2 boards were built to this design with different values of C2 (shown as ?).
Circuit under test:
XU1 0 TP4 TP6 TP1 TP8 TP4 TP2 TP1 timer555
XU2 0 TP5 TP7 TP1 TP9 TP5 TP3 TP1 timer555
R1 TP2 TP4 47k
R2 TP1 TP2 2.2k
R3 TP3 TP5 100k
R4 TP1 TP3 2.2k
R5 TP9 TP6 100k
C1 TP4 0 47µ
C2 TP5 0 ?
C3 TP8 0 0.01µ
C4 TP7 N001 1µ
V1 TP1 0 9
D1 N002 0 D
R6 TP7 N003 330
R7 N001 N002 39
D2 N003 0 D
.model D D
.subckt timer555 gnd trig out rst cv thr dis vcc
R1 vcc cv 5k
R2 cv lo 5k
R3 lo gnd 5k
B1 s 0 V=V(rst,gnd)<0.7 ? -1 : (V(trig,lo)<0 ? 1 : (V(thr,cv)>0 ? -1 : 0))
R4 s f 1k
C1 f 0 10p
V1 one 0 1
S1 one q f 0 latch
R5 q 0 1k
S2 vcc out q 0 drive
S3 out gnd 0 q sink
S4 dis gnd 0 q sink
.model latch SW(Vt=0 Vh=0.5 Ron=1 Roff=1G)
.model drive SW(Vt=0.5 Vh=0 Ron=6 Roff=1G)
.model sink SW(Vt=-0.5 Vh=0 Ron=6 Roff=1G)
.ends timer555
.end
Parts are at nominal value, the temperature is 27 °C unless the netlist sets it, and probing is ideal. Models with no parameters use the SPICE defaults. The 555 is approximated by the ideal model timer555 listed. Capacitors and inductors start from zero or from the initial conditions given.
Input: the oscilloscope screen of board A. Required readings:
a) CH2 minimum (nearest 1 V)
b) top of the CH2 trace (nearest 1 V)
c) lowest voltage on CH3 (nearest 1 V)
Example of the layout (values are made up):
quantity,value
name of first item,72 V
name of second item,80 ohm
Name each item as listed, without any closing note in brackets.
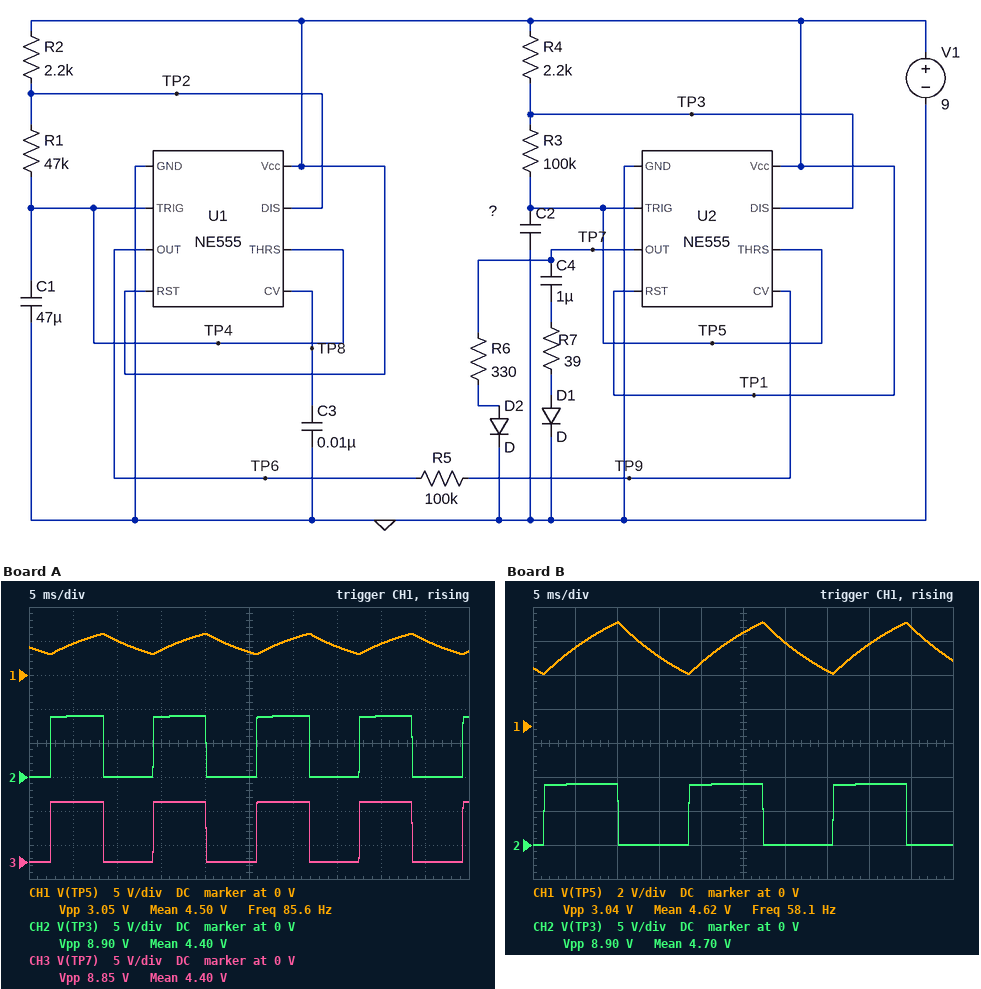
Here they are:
quantity,value
CH2 minimum,0 V
top of the CH2 trace,9 V
lowest voltage on CH3,0 V
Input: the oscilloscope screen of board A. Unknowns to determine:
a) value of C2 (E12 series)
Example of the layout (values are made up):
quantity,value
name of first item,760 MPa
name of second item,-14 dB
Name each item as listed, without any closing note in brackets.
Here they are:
quantity,value
value of C2,82 nF
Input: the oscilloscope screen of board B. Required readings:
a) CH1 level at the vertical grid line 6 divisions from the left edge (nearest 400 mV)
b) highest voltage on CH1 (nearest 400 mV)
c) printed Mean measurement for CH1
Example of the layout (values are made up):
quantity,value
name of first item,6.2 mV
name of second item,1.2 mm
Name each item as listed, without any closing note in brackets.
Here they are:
quantity,value
CH1 level at the vertical grid line 6 divisions from the left edge,4.8 V
highest voltage on CH1,6.0 V
printed Mean measurement for CH1,4.62 V
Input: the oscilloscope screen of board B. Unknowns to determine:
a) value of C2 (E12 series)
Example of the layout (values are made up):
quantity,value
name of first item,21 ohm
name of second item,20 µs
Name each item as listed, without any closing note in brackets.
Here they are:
quantity,value
value of C2,120 nF
